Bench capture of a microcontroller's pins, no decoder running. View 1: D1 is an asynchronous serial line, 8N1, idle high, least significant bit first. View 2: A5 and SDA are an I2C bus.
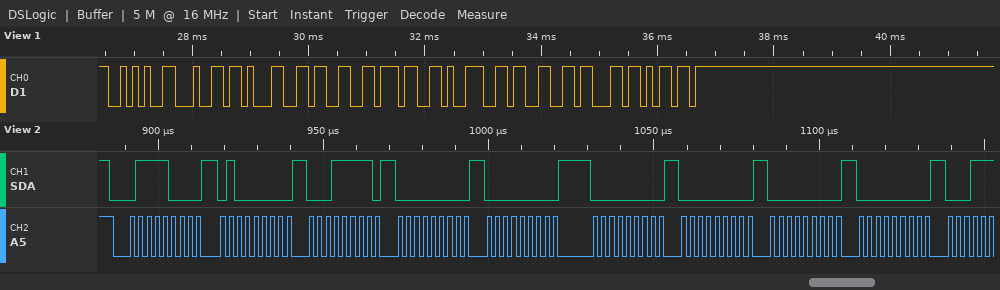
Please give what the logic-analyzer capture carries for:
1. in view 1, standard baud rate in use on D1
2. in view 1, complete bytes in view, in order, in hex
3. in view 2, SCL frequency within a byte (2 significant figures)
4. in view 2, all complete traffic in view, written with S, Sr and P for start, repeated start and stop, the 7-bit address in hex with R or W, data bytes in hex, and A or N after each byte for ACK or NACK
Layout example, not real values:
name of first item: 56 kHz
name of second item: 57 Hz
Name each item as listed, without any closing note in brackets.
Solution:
in view 1, standard baud rate in use on D1: 9600 baud
in view 1, complete bytes in view, in order, in hex: 0x2A 0x64 0x31 0x33 0x37 0x39 0x33 0x63 0x6D
in view 2, SCL frequency within a byte: 400 kHz
in view 2, all complete traffic in view, written with S, Sr and P for start, repeated start and stop, the 7-bit address in hex with R or W, data bytes in hex, and A or N after each byte for ACK or NACK: S 3CW A 40 A 1F A 00 A 00 A 00 A 00 A 00 A 00 A
